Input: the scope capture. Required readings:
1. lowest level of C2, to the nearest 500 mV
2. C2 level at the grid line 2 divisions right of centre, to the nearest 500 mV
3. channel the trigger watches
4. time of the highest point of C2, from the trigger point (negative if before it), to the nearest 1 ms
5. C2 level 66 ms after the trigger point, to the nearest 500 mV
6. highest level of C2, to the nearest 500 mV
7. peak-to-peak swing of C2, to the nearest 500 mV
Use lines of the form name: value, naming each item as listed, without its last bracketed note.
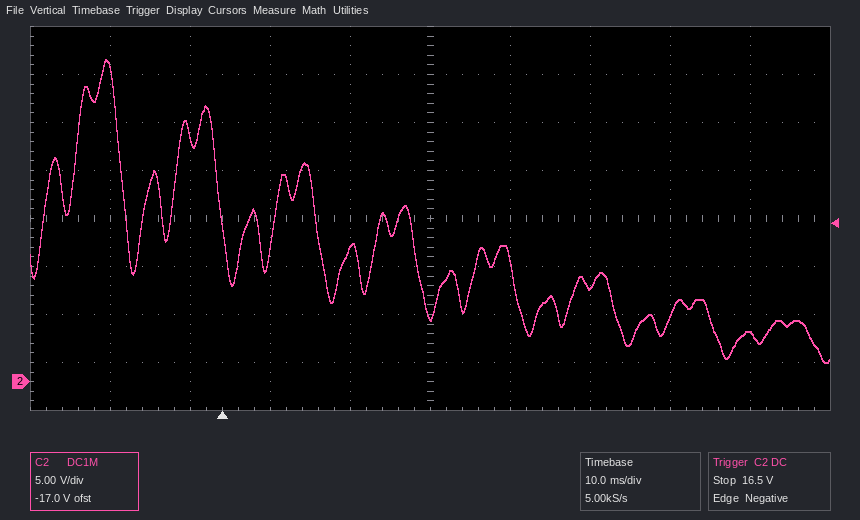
lowest level of C2, to the nearest 500 mV: 2.0 V
C2 level at the grid line 2 divisions right of centre, to the nearest 500 mV: 10.0 V
channel the trigger watches: C2
time of the highest point of C2, from the trigger point (negative if before it), to the nearest 1 ms: -14 ms
C2 level 66 ms after the trigger point, to the nearest 500 mV: 5.0 V
highest level of C2, to the nearest 500 mV: 33.5 V
peak-to-peak swing of C2, to the nearest 500 mV: 31.5 V
